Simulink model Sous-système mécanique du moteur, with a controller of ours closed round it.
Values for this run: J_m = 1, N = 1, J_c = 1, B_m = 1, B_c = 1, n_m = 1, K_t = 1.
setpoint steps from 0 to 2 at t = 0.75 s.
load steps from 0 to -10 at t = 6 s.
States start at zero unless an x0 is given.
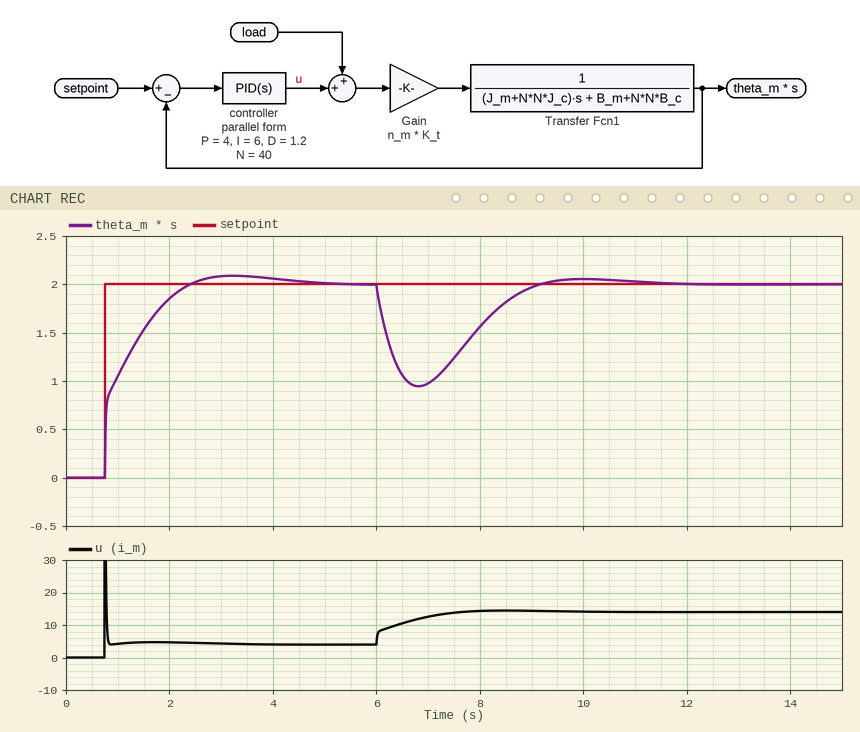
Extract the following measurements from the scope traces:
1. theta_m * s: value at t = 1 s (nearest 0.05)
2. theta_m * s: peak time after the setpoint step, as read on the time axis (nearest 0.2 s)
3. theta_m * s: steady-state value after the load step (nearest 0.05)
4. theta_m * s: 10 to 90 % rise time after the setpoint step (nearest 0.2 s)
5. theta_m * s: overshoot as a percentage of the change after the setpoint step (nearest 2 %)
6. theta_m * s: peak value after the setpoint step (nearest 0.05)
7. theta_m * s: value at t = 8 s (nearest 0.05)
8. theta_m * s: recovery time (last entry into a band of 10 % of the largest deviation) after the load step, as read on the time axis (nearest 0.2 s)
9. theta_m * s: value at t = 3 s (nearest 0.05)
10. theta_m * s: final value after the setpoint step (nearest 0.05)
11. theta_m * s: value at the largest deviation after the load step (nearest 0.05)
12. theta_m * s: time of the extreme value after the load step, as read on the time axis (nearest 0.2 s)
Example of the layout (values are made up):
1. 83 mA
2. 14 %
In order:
1. 1.05
2. 3.2 s
3. 2.00
4. 1.2 s
5. 4 %
6. 2.10
7. 1.55
8. 8.8 s
9. 2.10
10. 2.00
11. 0.95
12. 6.8 s
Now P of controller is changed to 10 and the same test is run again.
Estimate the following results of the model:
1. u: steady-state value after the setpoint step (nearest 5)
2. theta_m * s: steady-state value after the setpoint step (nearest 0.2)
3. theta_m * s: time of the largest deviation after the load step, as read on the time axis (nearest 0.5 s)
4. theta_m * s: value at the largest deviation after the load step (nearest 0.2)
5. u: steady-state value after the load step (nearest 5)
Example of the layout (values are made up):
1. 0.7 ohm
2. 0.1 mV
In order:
1. 5
2. 2.0
3. 6.5 s
4. 1.4
5. 15
